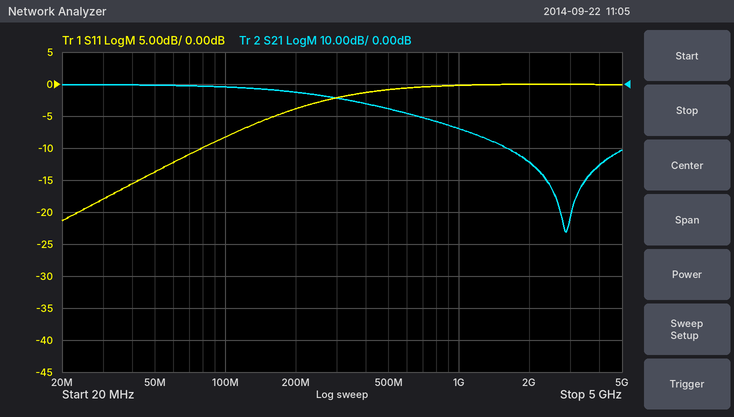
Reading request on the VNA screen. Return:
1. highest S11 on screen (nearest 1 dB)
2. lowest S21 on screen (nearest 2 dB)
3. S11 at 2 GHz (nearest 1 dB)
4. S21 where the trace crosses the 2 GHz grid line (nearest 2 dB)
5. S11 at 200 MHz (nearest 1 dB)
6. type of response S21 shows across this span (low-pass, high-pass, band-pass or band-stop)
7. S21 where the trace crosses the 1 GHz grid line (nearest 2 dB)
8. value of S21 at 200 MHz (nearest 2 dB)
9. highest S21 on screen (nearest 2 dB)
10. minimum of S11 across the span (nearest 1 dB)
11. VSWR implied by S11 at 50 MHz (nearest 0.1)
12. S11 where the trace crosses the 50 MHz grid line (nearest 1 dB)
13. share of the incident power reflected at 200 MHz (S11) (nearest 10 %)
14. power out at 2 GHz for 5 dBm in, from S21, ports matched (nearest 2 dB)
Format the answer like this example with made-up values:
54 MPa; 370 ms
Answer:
0 dB; -46 dB; 0 dB; -24 dB; -4 dB; low-pass; -14 dB; -2 dB; 0 dB; -21 dB; 1.5; -14 dB; 40 %; -20 dBm
